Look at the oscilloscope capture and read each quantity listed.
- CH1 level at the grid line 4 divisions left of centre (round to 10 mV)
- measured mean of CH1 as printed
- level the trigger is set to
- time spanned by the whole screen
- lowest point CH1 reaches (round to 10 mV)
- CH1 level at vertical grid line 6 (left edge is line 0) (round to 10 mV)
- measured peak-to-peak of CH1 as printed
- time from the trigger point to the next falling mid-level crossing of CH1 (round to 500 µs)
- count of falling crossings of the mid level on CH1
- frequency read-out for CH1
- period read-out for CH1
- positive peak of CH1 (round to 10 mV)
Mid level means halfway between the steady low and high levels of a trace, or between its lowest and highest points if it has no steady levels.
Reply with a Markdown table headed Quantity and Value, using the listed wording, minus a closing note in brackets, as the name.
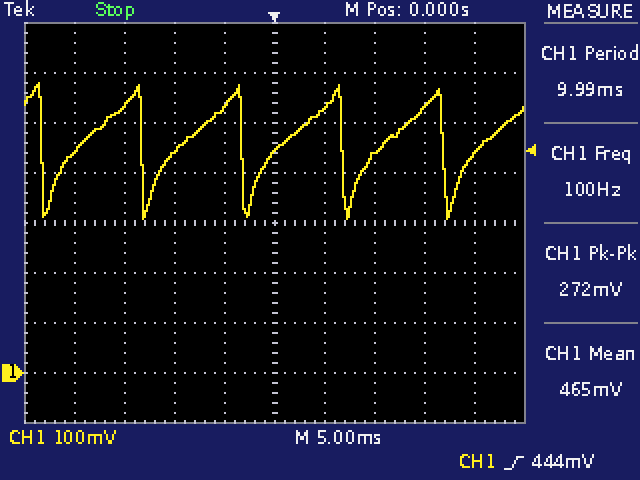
| Quantity | Value |
|---|---|
| CH1 level at the grid line 4 divisions left of centre | 440 mV |
| measured mean of CH1 as printed | 465 mV |
| level the trigger is set to | 444 mV |
| time spanned by the whole screen | 50 ms |
| lowest point CH1 reaches | 310 mV |
| CH1 level at vertical grid line 6 (left edge is line 0) | 530 mV |
| measured peak-to-peak of CH1 as printed | 272 mV |
| time from the trigger point to the next falling mid-level crossing of CH1 | 7.0 ms |
| count of falling crossings of the mid level on CH1 | 5 |
| frequency read-out for CH1 | 100 Hz |
| period read-out for CH1 | 9.99 ms |
| positive peak of CH1 | 580 mV |
